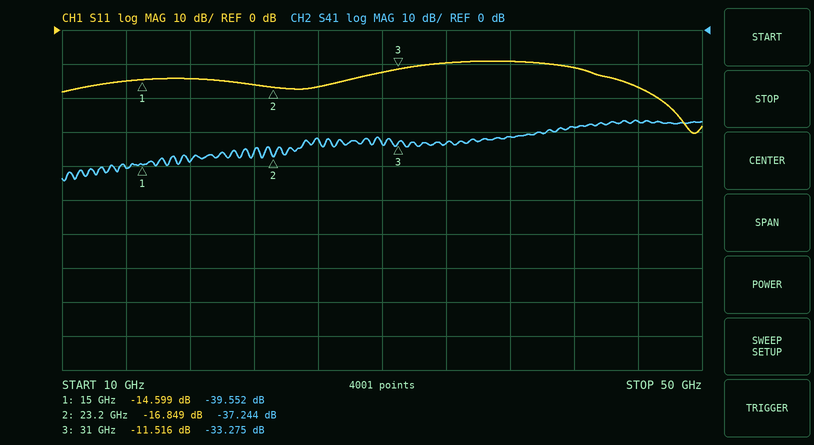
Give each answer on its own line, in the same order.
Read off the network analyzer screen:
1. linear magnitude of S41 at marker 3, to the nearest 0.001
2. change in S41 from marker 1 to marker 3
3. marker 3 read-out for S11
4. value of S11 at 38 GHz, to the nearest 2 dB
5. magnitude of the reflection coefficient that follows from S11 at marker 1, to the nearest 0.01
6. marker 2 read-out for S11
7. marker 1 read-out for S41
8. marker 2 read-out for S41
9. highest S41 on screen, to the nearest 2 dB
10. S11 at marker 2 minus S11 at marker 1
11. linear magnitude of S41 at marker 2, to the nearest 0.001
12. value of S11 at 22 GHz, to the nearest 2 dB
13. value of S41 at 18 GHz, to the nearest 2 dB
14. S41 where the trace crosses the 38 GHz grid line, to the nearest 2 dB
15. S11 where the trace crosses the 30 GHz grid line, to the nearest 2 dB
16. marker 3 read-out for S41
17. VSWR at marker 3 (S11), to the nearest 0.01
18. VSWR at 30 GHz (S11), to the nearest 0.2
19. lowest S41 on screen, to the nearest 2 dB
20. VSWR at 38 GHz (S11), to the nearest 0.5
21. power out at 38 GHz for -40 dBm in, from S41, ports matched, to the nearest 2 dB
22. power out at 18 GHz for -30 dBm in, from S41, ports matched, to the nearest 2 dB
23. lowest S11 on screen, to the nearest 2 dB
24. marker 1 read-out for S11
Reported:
0.022
6.277 dB
-11.516 dB
-10 dB
0.19
-16.849 dB
-39.552 dB
-37.244 dB
-26 dB
-2.250 dB
0.014
-16 dB
-38 dB
-32 dB
-12 dB
-33.275 dB
1.72
1.6
-44 dB
2.0
-72 dBm
-68 dBm
-30 dB
-14.599 dB
